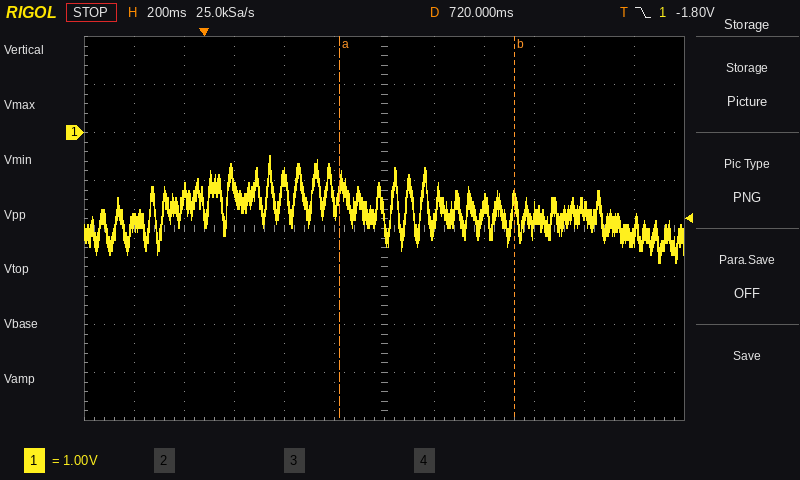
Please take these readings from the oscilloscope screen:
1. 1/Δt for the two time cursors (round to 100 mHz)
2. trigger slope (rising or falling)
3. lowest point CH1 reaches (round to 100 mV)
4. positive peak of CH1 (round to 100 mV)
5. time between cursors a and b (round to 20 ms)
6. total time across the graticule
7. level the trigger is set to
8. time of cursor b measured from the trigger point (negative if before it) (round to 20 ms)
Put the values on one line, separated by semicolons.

1.4 Hz; falling; -2.7 V; -500 mV; 700 ms; 2.4 s; -1.80 V; +1.24 s
